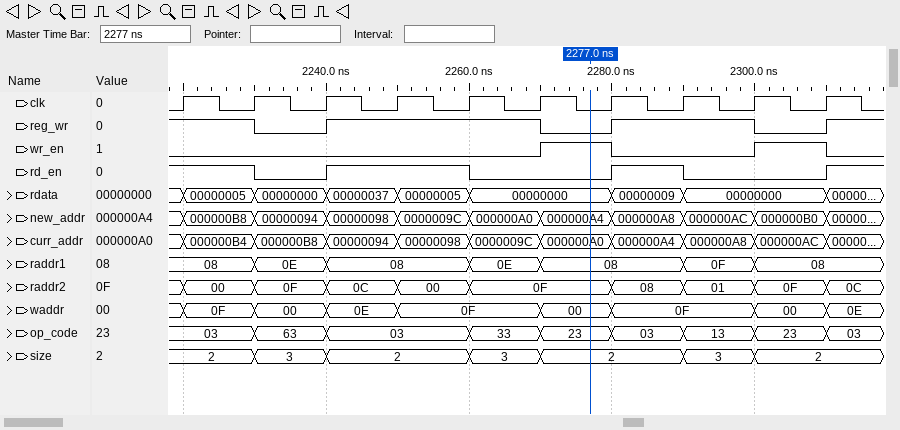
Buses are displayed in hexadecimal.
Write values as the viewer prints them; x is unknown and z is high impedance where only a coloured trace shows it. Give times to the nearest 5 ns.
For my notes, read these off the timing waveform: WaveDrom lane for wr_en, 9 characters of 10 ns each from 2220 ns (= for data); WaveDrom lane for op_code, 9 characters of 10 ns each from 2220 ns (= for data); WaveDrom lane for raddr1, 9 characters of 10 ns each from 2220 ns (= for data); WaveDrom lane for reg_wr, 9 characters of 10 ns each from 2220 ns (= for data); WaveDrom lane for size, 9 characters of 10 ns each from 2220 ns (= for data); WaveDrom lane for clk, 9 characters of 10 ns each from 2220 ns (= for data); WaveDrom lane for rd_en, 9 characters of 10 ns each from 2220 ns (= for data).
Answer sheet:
{name: 'wr_en', wave: '0....10.1'}
{name: 'op_code', wave: '===.=====', data: '03 63 03 33 23 03 13 23'}
{name: 'raddr1', wave: '===.==.==', data: '08 0E 08 0E 08 0F 08'}
{name: 'reg_wr', wave: '101..01.0'}
{name: 'size', wave: '===.==.==', data: '2 3 2 3 2 3 2'}
{name: 'clk', wave: 'p........'}
{name: 'rd_en', wave: '101.0.10.'}
